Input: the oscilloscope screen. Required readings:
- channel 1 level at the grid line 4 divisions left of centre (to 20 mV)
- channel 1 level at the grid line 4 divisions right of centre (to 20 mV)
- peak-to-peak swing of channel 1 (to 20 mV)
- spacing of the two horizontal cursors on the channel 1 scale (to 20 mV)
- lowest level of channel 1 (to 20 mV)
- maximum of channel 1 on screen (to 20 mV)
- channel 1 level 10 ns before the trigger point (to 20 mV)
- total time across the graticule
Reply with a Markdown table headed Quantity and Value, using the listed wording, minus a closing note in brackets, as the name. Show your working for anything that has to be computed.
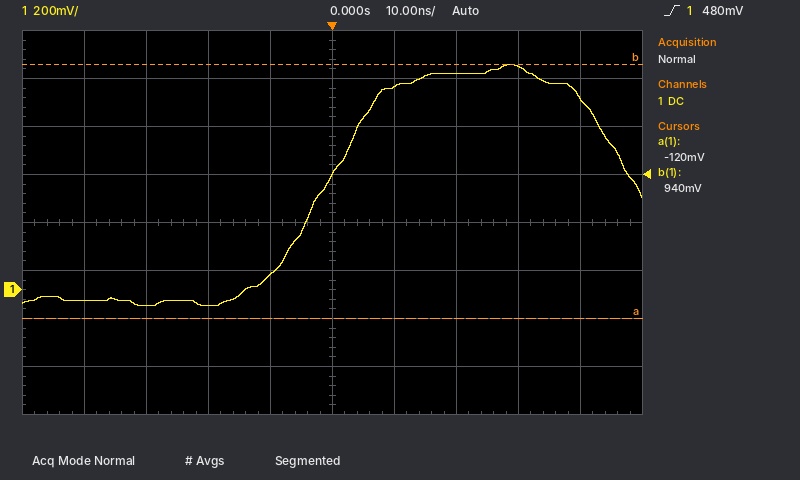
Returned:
| Quantity | Value |
|---|---|
| channel 1 level at the grid line 4 divisions left of centre | -40 mV |
| channel 1 level at the grid line 4 divisions right of centre | 800 mV |
| peak-to-peak swing of channel 1 | 940 mV − (-60 mV) = 1.00 V |
| spacing of the two horizontal cursors on the channel 1 scale | 1.06 V |
| lowest level of channel 1 | -60 mV |
| maximum of channel 1 on screen | 940 mV |
| channel 1 level 10 ns before the trigger point | 60 mV |
| total time across the graticule | 100 ns |
